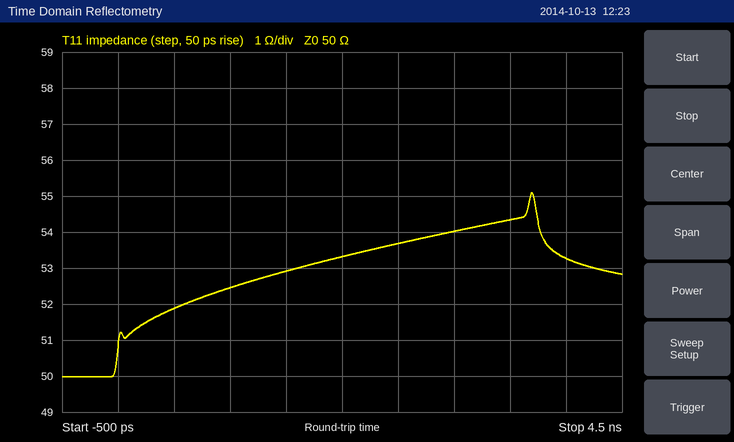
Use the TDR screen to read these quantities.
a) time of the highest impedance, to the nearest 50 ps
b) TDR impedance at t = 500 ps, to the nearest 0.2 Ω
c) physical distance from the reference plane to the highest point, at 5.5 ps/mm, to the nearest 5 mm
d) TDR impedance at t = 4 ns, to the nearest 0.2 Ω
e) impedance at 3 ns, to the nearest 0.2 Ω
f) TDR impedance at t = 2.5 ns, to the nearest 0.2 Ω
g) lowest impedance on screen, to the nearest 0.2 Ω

3.70 ns
51.8 Ω
335 mm
53.2 Ω
54.0 Ω
53.6 Ω
50.0 Ω
